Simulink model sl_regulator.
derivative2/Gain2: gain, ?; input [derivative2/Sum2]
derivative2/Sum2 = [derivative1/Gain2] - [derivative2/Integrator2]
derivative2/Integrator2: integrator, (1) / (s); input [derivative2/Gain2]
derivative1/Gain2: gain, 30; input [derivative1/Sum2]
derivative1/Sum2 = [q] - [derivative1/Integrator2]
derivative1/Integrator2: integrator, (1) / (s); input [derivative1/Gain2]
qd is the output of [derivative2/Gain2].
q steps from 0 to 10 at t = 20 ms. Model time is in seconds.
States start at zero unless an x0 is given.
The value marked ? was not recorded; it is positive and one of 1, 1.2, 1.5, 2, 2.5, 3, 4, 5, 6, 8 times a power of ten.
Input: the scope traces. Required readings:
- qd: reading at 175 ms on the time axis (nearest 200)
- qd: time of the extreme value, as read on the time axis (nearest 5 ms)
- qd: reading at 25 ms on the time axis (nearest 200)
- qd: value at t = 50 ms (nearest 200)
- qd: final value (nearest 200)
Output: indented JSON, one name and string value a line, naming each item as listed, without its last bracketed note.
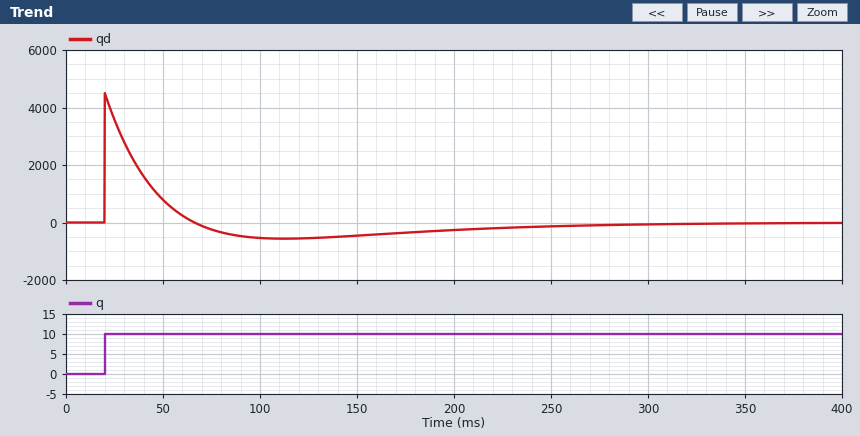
{
  "qd: reading at 175 ms on the time axis": "-400",
  "qd: time of the extreme value, as read on the time axis": "20 ms",
  "qd: reading at 25 ms on the time axis": "3600",
  "qd: value at t = 50 ms": "800",
  "qd: final value": "0"
}
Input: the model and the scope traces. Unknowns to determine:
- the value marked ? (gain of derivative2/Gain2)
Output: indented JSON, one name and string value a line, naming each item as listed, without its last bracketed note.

{
  "the value marked ?": "15"
}
